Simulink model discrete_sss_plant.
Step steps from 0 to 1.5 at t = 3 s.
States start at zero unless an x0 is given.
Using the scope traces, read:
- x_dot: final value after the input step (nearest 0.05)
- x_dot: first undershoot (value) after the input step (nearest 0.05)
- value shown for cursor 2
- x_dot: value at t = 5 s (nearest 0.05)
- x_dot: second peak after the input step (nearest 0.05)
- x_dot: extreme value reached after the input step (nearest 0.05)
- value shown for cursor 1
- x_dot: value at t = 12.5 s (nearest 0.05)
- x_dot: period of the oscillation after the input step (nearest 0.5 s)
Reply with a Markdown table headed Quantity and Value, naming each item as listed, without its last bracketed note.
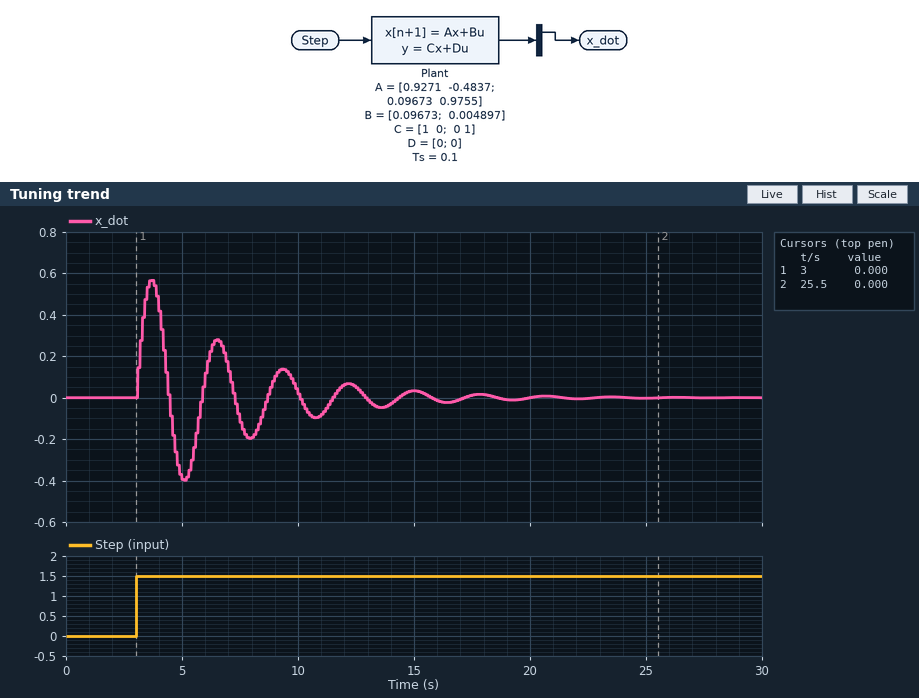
| Quantity | Value |
|---|---|
| x_dot: final value after the input step | 0.00 |
| x_dot: first undershoot (value) after the input step | -0.40 |
| value shown for cursor 2 | 0.000 |
| x_dot: value at t = 5 s | -0.40 |
| x_dot: second peak after the input step | 0.30 |
| x_dot: extreme value reached after the input step | 0.55 |
| value shown for cursor 1 | 0.000 |
| x_dot: value at t = 12.5 s | 0.05 |
| x_dot: period of the oscillation after the input step | 3.0 s |
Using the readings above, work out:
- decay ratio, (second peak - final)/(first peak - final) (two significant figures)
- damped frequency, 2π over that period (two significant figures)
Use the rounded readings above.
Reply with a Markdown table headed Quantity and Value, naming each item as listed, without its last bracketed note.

| Quantity | Value |
|---|---|
| decay ratio, (second peak - final)/(first peak - final) | 0.55 |
| damped frequency, 2π over that period | 2.1 rad/s |
